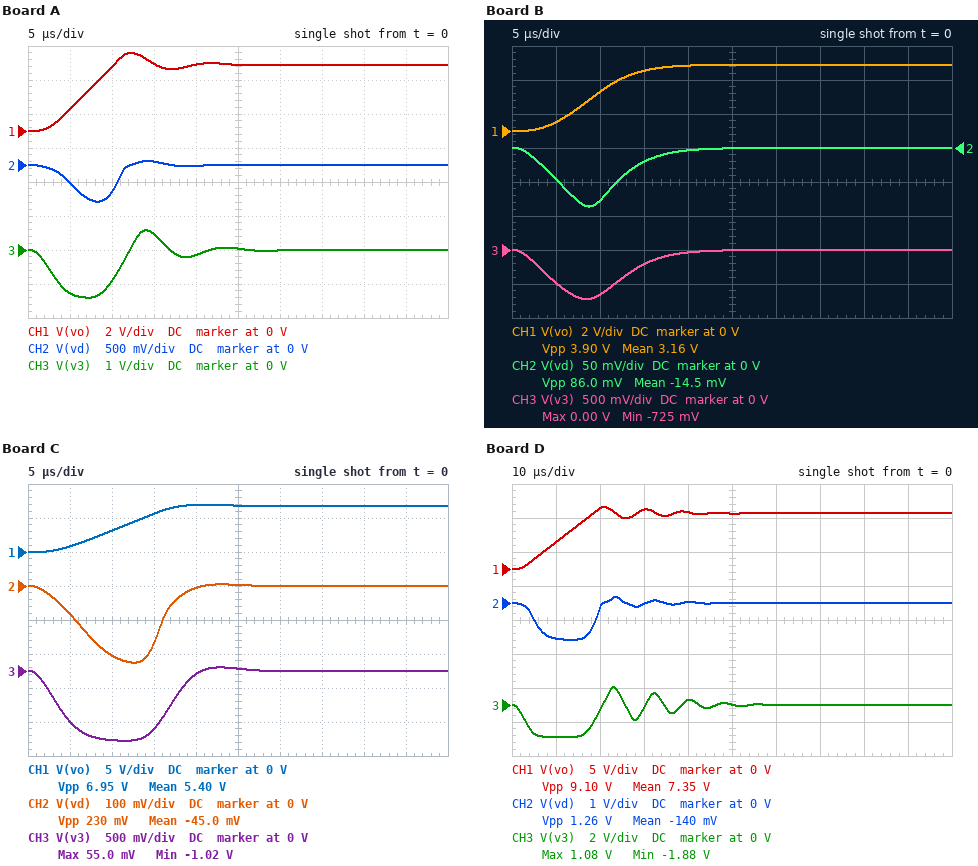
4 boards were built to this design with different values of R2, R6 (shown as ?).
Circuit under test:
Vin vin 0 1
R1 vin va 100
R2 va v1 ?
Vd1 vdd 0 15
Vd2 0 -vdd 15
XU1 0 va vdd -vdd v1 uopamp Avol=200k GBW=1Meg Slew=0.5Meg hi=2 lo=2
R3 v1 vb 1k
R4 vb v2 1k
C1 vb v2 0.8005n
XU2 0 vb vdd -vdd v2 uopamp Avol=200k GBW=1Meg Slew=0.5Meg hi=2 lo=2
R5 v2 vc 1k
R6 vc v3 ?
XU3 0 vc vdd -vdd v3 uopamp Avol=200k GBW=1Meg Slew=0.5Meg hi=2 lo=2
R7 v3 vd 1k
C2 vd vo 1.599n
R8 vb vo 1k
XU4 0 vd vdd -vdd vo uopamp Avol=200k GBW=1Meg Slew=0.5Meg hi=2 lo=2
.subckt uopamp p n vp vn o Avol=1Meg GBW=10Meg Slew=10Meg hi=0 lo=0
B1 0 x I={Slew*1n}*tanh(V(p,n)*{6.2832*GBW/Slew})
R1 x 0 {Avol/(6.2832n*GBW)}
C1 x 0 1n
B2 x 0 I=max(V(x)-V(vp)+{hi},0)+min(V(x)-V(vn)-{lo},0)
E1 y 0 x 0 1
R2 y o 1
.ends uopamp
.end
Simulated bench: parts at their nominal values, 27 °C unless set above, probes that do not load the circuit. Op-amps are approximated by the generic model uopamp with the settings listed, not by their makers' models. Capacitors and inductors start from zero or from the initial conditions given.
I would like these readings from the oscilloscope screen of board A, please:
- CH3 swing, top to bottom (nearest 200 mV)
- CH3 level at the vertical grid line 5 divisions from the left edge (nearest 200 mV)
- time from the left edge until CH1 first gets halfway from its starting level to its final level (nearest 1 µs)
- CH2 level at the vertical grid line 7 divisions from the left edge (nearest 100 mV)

2.0 V
0 V
6 µs
0 V
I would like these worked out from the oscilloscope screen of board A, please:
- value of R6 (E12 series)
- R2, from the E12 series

1.2 kΩ
390 Ω
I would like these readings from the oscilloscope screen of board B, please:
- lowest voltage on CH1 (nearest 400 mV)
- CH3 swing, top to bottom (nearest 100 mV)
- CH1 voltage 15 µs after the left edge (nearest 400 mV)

0 V
700 mV
3.6 V
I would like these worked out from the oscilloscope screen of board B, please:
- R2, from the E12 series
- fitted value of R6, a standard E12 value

390 Ω
330 Ω
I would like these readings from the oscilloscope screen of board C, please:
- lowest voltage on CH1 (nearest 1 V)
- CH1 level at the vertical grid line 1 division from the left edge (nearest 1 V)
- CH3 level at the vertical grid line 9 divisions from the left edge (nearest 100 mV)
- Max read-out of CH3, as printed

0 V
1 V
0 V
55.0 mV
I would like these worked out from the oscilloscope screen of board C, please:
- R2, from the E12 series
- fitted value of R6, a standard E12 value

680 Ω
560 Ω
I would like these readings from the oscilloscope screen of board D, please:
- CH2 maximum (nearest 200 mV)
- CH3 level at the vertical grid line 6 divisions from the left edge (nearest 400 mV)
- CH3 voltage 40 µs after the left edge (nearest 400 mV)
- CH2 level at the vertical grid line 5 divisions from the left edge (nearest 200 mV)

200 mV
0 V
400 mV
0 V
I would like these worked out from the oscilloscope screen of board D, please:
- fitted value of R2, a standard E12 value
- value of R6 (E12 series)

820 Ω
1.8 kΩ
